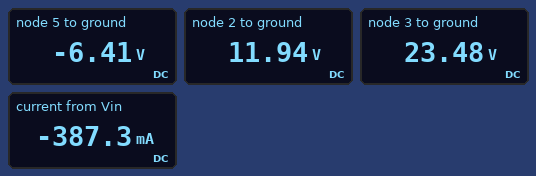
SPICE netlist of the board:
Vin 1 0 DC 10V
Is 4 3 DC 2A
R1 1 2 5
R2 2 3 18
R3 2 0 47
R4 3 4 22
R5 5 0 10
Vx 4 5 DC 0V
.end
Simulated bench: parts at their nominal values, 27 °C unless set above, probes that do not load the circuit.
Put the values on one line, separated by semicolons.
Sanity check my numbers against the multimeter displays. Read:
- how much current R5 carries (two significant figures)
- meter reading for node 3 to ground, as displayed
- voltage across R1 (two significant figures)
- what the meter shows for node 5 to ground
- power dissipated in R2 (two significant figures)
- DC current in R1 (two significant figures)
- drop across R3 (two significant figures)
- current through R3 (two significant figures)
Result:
640 mA; 23.48 V; 1.9 V; -6.41 V; 7.4 W; 390 mA; 12 V; 250 mA
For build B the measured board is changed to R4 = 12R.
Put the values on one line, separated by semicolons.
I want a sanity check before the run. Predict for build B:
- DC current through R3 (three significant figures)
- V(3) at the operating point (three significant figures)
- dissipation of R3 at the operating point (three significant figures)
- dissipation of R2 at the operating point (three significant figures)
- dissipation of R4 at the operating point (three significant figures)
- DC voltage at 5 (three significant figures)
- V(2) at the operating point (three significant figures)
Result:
225 mA; 16.6 V; 2.37 W; 2.03 W; 33.2 W; -3.36 V; 10.6 V
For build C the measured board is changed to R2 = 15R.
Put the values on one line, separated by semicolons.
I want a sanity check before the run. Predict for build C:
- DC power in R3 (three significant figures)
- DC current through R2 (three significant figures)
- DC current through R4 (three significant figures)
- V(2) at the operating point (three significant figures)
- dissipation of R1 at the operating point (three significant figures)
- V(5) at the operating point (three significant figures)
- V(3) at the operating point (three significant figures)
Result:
3.12 W; 679 mA; 1.32 A; 12.1 V; 886 mW; -6.79 V; 22.3 V
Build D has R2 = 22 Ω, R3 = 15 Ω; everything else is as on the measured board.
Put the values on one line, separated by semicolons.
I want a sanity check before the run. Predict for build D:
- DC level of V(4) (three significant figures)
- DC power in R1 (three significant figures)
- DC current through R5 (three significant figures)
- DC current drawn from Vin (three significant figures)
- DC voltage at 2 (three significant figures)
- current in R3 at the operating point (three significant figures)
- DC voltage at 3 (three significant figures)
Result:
-6.32 V; 3.37 mW; 632 mA; 26.0 mA; 9.87 V; 658 mA; 23.8 V
